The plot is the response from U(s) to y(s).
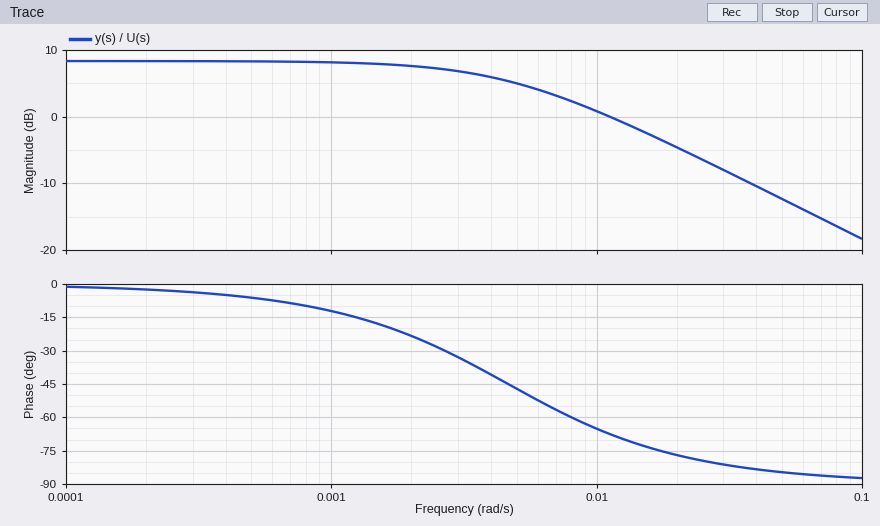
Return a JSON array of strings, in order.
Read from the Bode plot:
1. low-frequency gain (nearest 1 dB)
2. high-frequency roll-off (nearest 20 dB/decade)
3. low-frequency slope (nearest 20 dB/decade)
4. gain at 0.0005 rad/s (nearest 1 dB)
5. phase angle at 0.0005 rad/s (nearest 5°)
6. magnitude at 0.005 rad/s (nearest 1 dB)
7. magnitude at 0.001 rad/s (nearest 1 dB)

["8 dB", "-20 dB/decade", "0 dB/decade", "8 dB", "-5°", "5 dB", "8 dB"]
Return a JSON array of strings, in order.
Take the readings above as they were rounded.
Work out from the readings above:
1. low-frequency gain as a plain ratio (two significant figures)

["2.5"]
